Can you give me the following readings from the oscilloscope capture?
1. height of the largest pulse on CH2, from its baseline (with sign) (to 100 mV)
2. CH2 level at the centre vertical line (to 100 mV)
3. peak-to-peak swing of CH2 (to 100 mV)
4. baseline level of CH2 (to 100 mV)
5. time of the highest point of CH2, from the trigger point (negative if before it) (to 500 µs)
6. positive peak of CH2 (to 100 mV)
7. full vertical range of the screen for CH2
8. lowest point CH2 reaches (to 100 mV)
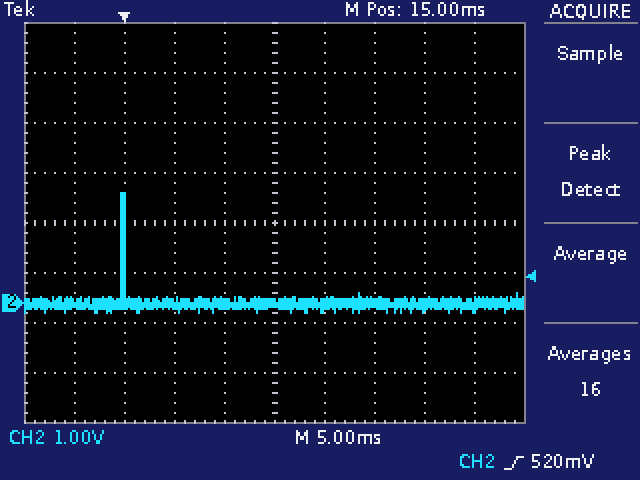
+2.2 V
0.0 V
2.4 V
0.0 V
0.0 ms
2.2 V
8 V
-200 mV
